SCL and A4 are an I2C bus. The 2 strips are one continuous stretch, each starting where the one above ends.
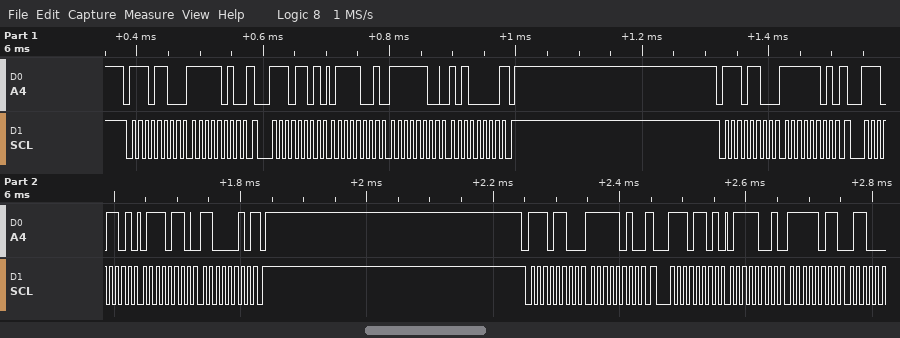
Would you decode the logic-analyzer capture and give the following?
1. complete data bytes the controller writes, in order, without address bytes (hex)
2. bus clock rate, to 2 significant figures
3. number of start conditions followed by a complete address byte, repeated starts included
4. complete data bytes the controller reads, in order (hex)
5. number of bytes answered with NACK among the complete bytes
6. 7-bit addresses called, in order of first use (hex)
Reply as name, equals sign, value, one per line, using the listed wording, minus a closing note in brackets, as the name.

complete data bytes the controller writes, in order, without address bytes = FA FD FA
bus clock rate, to 2 significant figures = 100 kHz
number of start conditions followed by a complete address byte, repeated starts included = 6
complete data bytes the controller reads, in order = 79 FC A0 76 C2 79 FB
number of bytes answered with NACK among the complete bytes = 2
7-bit addresses called, in order of first use = 0x76
